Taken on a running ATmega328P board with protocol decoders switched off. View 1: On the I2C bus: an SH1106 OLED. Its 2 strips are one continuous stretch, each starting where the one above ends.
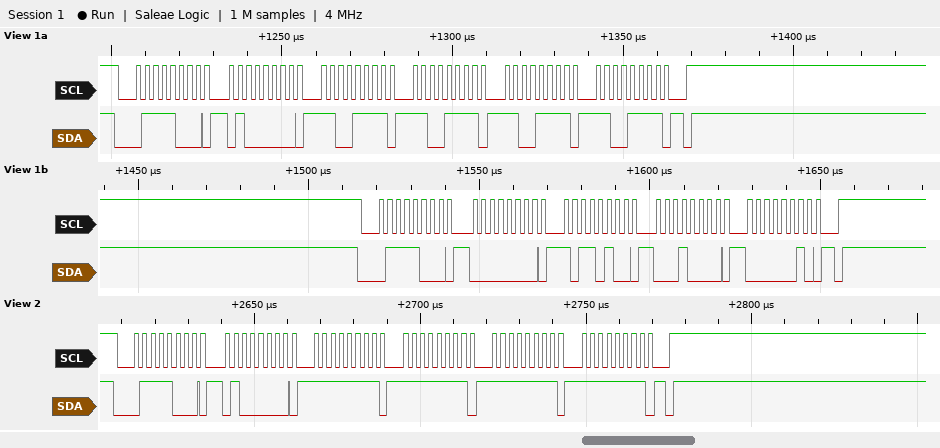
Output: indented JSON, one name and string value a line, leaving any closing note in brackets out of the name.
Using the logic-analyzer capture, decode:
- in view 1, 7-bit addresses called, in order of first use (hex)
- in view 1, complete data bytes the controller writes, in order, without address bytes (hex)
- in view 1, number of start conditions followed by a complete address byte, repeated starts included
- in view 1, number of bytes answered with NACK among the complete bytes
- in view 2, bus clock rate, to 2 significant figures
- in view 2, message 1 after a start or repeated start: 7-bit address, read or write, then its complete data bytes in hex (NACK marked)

{
  "in view 1, 7-bit addresses called, in order of first use": "0x3C",
  "in view 1, complete data bytes the controller writes, in order, without address bytes": "40 CF CF CF CF 00 B4 10 02",
  "in view 1, number of start conditions followed by a complete address byte, repeated starts included": "2",
  "in view 1, number of bytes answered with NACK among the complete bytes": "0",
  "in view 2, bus clock rate, to 2 significant figures": "400 kHz",
  "in view 2, message 1 after a start or repeated start: 7-bit address, read or write, then its complete data bytes in hex": "0x3C write: 40 FF FF FF FF"
}
